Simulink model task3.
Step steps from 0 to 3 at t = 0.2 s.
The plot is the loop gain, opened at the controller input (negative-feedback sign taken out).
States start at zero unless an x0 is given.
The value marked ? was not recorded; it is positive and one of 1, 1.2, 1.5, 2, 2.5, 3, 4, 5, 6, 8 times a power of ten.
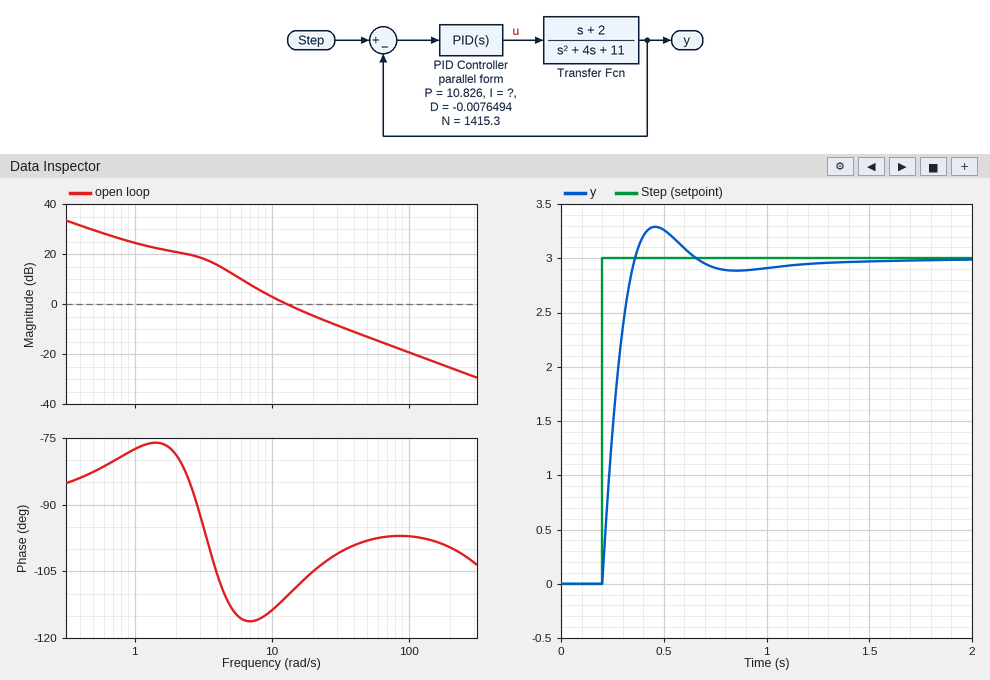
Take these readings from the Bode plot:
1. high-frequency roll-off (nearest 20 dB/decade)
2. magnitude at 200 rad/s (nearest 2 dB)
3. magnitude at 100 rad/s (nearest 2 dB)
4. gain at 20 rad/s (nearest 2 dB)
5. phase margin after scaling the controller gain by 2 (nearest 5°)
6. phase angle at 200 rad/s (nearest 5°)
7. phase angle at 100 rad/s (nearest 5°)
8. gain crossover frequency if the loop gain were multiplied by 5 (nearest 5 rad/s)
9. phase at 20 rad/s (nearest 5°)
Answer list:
-20 dB/decade
-26 dB
-20 dB
-4 dB
75°
-100°
-95°
55 rad/s
-105°
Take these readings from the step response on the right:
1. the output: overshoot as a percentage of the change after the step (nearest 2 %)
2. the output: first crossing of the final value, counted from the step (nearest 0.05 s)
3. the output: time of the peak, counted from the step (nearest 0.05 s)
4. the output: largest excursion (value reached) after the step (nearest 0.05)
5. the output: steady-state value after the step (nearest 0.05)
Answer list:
10 %
0.15 s
0.25 s
3.30
3.00
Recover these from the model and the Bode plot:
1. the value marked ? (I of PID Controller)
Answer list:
80
